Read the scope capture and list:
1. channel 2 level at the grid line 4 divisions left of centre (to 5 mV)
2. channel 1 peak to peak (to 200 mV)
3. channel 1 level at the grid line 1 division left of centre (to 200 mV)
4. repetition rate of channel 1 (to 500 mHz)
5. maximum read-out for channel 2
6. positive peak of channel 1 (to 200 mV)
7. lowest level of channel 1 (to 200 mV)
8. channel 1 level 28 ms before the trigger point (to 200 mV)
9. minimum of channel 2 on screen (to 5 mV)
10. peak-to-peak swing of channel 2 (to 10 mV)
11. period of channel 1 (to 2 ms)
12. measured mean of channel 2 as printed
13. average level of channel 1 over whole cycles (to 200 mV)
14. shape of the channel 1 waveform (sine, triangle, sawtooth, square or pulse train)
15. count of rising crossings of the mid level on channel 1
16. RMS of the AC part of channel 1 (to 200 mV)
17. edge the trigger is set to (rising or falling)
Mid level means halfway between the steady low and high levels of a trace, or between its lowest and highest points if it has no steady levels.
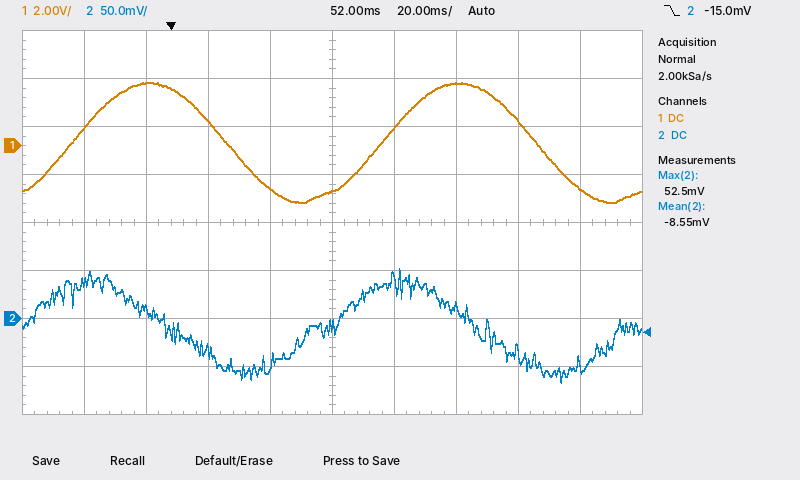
40 mV
5.0 V
-1.8 V
10.0 Hz
52.5 mV
2.6 V
-2.4 V
800 mV
-65 mV
120 mV
100 ms
-8.55 mV
200 mV
sine
2
1.8 V
falling
